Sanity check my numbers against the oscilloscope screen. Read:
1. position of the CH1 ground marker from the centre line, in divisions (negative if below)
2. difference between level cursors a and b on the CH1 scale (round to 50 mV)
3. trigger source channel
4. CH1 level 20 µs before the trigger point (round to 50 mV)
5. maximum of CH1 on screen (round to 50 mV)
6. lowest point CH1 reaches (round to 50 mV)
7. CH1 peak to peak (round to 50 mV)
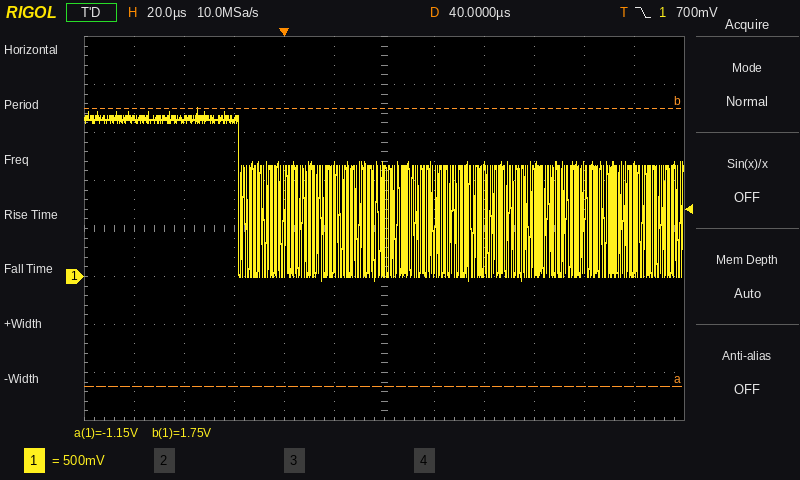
-1.0 div
2.90 V
CH1
1.65 V
1.75 V
-50 mV
1.80 V
